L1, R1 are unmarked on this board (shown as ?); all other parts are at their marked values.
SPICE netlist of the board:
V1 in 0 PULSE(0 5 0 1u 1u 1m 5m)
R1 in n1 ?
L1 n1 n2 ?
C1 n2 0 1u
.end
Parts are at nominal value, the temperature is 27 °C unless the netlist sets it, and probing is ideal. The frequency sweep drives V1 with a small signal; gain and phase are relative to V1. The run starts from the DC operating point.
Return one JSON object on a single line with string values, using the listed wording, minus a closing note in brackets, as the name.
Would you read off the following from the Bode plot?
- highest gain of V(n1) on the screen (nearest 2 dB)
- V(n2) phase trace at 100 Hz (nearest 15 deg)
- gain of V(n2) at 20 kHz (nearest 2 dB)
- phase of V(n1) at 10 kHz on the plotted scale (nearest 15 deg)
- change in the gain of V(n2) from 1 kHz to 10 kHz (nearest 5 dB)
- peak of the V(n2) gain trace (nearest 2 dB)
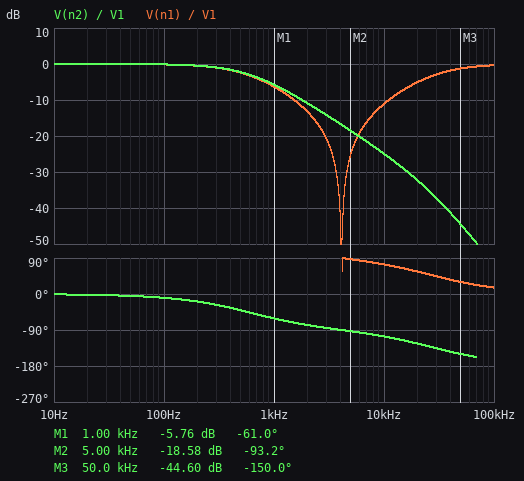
{"highest gain of V(n1) on the screen": "0 dB", "V(n2) phase trace at 100 Hz": "-15 deg", "gain of V(n2) at 20 kHz": "-32 dB", "phase of V(n1) at 10 kHz on the plotted scale": "75 deg", "change in the gain of V(n2) from 1 kHz to 10 kHz": "-20 dB", "peak of the V(n2) gain trace": "0 dB"}
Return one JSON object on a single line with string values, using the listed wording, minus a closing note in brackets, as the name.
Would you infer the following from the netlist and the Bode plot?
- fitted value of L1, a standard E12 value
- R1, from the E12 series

{"fitted value of L1, a standard E12 value": "1.5 mH", "R1, from the E12 series": "270 Ω"}
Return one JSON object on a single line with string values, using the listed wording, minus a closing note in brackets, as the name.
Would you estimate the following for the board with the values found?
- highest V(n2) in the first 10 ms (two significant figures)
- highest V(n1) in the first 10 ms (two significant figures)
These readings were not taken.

{"highest V(n2) in the first 10 ms": "4.9 V", "highest V(n1) in the first 10 ms": "4.9 V"}
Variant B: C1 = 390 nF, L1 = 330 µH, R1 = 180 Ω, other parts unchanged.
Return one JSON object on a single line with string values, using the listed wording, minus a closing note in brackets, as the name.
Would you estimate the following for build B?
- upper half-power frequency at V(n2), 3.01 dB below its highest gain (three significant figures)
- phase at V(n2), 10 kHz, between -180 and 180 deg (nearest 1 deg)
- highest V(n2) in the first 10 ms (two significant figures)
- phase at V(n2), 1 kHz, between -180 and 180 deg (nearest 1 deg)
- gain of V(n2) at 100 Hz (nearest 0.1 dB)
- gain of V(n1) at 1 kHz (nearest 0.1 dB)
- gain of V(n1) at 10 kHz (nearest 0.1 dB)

{"upper half-power frequency at V(n2), 3.01 dB below its highest gain": "2.33 kHz", "phase at V(n2), 10 kHz, between -180 and 180 deg": "-84 deg", "highest V(n2) in the first 10 ms": "5.0 V", "phase at V(n2), 1 kHz, between -180 and 180 deg": "-24 deg", "gain of V(n2) at 100 Hz": "0 dB", "gain of V(n1) at 1 kHz": "-0.8 dB", "gain of V(n1) at 10 kHz": "-19.1 dB"}
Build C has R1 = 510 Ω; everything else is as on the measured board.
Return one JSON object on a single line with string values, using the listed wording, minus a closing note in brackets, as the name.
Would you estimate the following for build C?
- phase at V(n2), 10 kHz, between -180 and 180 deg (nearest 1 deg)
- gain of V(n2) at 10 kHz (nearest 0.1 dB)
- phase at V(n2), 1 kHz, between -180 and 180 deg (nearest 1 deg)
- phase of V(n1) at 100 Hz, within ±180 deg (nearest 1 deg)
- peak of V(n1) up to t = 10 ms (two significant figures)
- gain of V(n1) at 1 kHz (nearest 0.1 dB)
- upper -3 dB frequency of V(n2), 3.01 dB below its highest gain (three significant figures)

{"phase at V(n2), 10 kHz, between -180 and 180 deg": "-99 deg", "gain of V(n2) at 10 kHz": "-30.2 dB", "phase at V(n2), 1 kHz, between -180 and 180 deg": "-74 deg", "phase of V(n1) at 100 Hz, within ±180 deg": "-18 deg", "peak of V(n1) up to t = 10 ms": "4.3 V", "gain of V(n1) at 1 kHz": "-11.0 dB", "upper -3 dB frequency of V(n2), 3.01 dB below its highest gain": "314 Hz"}
